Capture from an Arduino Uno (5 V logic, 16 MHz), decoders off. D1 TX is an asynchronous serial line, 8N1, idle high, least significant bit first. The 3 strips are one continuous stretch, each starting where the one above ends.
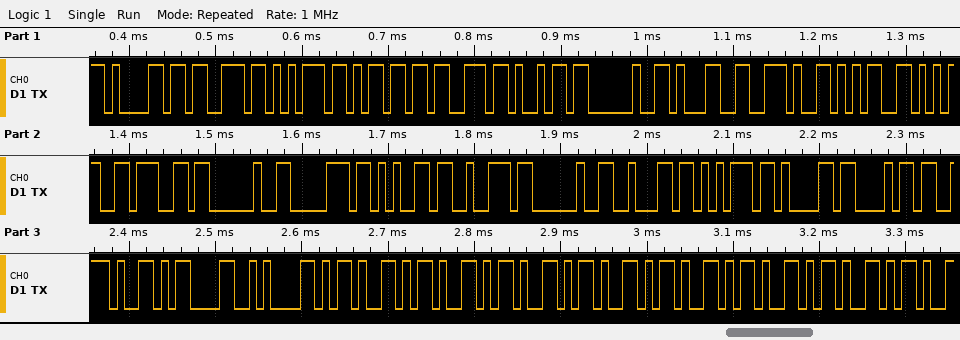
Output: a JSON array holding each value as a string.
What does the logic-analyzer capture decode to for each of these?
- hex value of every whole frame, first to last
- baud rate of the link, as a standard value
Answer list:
["0x61 0x73 0x75 0x6D 0x73 0x69 0x20 0x31 0x2E 0x35 0x35 0x67 0x20 0x70 0x65 0x72 0x20 0x62 0x75 0x61 0x68 0x2E 0x0D 0x0A 0x2D 0x2D 0x2D 0x2D 0x2D 0x2D 0x2D 0x2D", "115200 baud"]
